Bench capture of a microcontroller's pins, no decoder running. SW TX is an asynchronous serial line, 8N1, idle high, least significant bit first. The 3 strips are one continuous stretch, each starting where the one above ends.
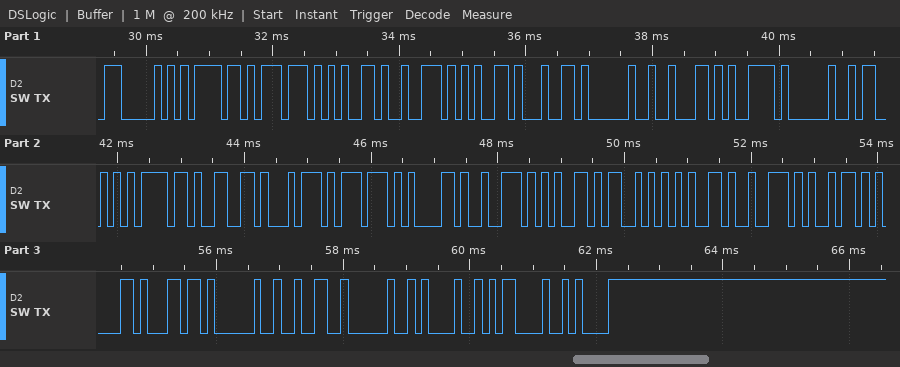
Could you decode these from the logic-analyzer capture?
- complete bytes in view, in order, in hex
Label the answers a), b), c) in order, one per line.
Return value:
a) 0x50 0x6F 0x77 0x65 0x72 0x65 0x64 0x20 0x62 0x79 0x20 0x53 0x6F 0x66 0x74 0x77 0x61 0x72 0x65 0x53 0x65 0x72 0x69 0x61 0x6C 0x20 0x32 0x20 0x21 0x0D 0x0A
